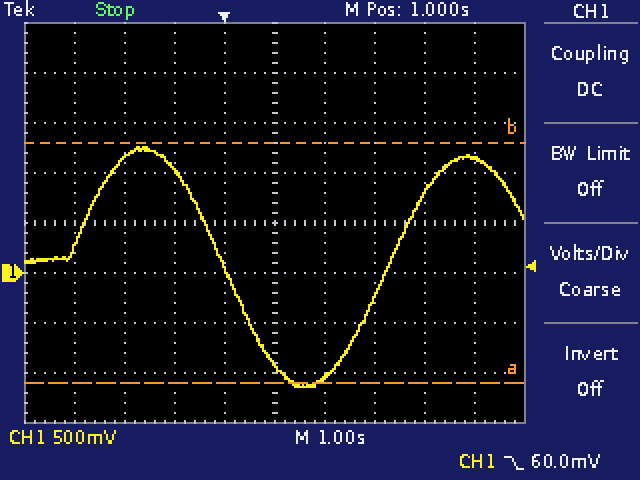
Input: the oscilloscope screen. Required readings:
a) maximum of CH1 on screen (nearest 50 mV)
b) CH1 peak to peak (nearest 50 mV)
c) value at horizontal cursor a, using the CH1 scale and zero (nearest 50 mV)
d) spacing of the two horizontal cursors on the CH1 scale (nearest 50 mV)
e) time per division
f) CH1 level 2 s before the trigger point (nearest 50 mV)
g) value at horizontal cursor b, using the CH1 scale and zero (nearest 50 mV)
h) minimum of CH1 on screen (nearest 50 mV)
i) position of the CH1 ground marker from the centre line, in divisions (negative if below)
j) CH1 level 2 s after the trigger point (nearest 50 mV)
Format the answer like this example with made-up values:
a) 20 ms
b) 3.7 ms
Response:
a) 1.25 V
b) 2.40 V
c) -1.10 V
d) 2.40 V
e) 1 s
f) 1.15 V
g) 1.30 V
h) -1.15 V
i) -1.0 div
j) -1.05 V
